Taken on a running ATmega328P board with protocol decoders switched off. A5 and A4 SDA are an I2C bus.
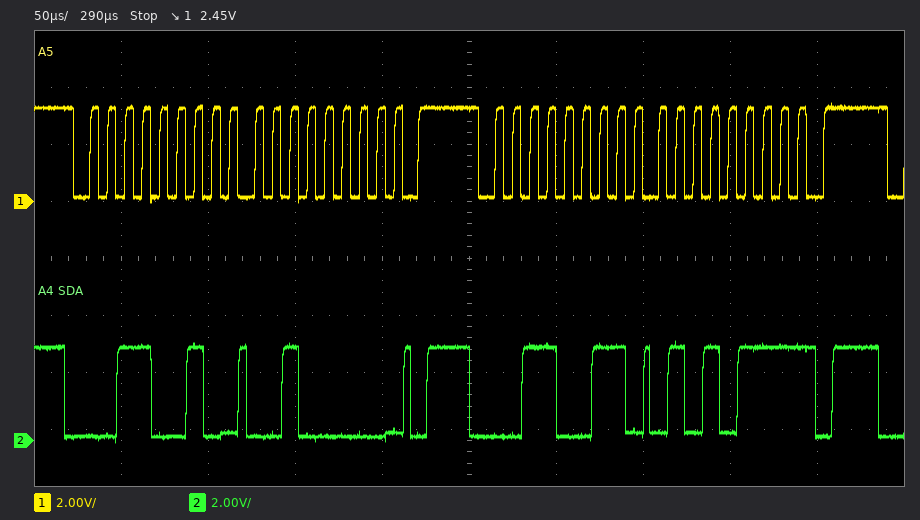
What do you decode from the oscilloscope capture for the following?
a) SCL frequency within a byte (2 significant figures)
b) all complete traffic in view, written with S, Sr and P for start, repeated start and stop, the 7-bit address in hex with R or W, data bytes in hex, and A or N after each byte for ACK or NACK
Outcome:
100 kHz
S 19W A 20 A P S 19R A 57 N P
